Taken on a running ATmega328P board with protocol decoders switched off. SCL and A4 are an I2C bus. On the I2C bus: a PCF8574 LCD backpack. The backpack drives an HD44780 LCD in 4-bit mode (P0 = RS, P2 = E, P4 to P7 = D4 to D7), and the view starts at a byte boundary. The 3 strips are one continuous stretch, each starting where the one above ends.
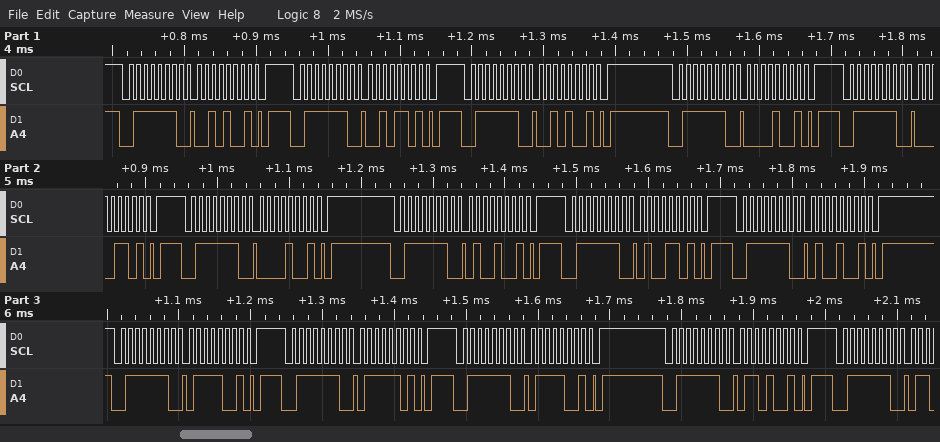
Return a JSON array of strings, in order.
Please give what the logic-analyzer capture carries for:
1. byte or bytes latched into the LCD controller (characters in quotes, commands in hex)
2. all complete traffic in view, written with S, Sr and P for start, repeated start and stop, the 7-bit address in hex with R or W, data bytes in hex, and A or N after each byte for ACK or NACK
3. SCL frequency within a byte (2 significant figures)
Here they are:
["' ' 'G'", "S 3FW A 29 A P S 3FW A 2D A P S 3FW A 29 A P S 3FW A 09 A P S 3FW A 0D A P S 3FW A 09 A P S 3FW A 49 A P S 3FW A 4D A P S 3FW A 49 A P S 3FW A 79 A P S 3FW A 7D A P S 3FW A 79 A P S 3FW A 69 A P S 3FW A", "100 kHz"]
